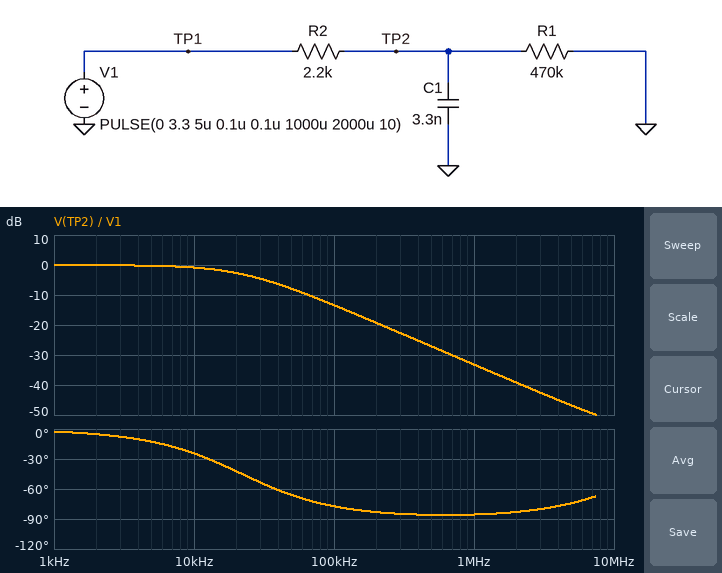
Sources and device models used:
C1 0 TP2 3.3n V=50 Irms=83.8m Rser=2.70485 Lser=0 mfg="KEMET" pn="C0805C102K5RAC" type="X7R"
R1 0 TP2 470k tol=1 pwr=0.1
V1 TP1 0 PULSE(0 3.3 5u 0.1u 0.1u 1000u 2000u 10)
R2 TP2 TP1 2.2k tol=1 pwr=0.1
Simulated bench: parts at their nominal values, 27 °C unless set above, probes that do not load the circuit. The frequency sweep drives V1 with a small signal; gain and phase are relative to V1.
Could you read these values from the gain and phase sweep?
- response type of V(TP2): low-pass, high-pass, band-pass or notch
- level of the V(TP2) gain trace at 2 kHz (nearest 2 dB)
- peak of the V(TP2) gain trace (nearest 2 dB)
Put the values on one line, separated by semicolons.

low-pass; 0 dB; 0 dB
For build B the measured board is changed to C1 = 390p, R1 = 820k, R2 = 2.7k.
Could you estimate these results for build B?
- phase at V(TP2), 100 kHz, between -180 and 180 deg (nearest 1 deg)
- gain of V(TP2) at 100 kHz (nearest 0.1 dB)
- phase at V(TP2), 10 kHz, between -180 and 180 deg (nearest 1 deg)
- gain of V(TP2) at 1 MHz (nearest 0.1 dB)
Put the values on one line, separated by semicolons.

-33 deg; -1.6 dB; -4 deg; -16.5 dB
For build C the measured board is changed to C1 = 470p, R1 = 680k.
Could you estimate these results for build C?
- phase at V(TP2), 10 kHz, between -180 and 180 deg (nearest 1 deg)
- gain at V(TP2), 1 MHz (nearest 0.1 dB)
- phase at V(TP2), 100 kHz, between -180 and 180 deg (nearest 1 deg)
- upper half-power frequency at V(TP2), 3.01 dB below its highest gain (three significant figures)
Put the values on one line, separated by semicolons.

-4 deg; -16.4 dB; -33 deg; 154 kHz
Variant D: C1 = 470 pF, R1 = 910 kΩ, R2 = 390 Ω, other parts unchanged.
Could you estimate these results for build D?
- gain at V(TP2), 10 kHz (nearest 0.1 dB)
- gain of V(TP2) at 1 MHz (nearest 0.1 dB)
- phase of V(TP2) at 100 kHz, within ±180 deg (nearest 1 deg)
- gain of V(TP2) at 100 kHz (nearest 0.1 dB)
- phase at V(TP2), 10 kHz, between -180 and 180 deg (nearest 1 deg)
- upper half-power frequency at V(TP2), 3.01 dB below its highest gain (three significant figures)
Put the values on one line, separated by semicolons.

0 dB; -3.7 dB; -7 deg; -0.1 dB; -1 deg; 863 kHz
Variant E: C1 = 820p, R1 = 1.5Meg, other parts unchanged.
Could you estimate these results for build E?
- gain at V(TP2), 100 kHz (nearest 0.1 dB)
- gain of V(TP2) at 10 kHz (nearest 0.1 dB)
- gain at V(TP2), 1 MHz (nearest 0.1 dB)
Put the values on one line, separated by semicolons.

-3.6 dB; -0.1 dB; -21.1 dB
